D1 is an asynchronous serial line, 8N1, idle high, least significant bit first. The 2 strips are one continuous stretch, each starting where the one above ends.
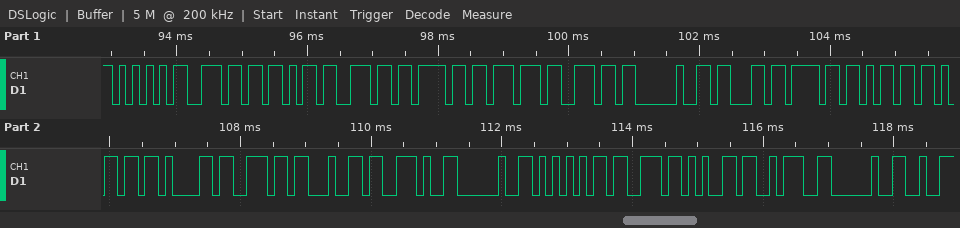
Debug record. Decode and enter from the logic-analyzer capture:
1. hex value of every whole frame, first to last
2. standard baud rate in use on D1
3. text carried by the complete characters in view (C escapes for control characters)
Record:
0x55 0x6E 0x6B 0x6E 0x6F 0x77 0x6E 0x20 0x63 0x6F 0x6D 0x6D 0x61 0x6E 0x64 0x2E 0x20 0x55 0x73 0x65 0x3A 0x20
9600 baud
"Unknown command. Use: "
